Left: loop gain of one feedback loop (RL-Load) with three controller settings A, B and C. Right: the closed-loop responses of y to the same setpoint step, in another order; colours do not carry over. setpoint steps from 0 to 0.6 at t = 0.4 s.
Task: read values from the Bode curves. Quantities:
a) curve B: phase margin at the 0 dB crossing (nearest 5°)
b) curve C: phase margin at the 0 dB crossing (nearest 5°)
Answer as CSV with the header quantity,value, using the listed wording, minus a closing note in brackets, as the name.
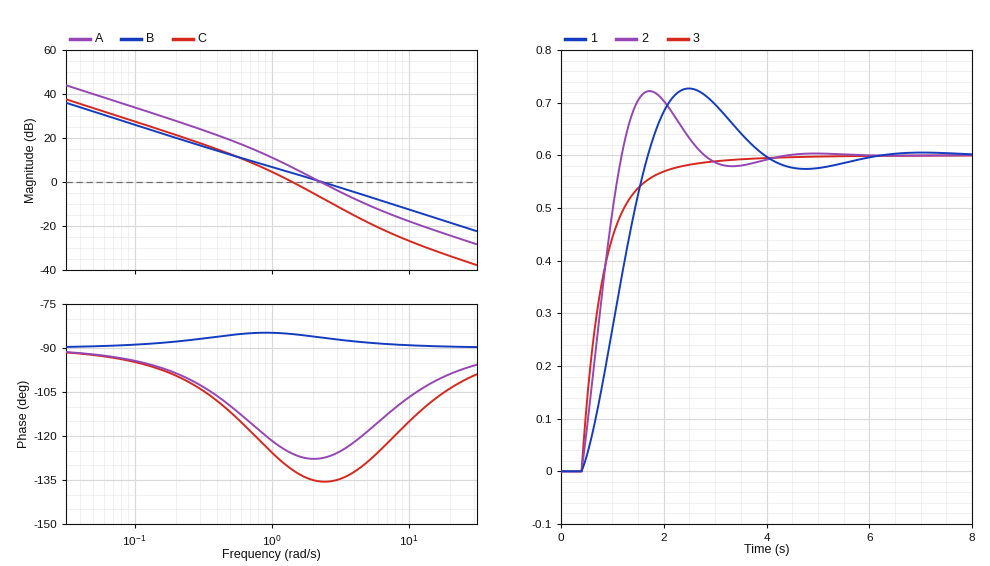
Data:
quantity,value
curve B: phase margin at the 0 dB crossing,95°
curve C: phase margin at the 0 dB crossing,50°
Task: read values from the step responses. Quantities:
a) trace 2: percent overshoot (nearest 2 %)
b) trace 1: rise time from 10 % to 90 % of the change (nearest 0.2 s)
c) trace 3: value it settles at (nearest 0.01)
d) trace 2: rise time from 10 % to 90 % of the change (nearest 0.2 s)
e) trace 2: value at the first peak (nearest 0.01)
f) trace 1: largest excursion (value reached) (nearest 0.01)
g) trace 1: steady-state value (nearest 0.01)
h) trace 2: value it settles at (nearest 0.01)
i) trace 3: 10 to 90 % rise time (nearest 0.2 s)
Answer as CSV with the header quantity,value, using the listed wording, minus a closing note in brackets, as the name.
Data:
quantity,value
trace 2: percent overshoot,20 %
trace 1: rise time from 10 % to 90 % of the change,1.0 s
trace 3: value it settles at,0.60
trace 2: rise time from 10 % to 90 % of the change,0.6 s
trace 2: value at the first peak,0.72
trace 1: largest excursion (value reached),0.73
trace 1: steady-state value,0.60
trace 2: value it settles at,0.60
trace 3: 10 to 90 % rise time,1.0 s
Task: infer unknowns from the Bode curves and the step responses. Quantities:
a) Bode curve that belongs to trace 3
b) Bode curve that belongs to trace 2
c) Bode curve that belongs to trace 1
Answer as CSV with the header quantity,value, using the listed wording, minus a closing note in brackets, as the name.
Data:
quantity,value
Bode curve that belongs to trace 3,B
Bode curve that belongs to trace 2,A
Bode curve that belongs to trace 1,C
